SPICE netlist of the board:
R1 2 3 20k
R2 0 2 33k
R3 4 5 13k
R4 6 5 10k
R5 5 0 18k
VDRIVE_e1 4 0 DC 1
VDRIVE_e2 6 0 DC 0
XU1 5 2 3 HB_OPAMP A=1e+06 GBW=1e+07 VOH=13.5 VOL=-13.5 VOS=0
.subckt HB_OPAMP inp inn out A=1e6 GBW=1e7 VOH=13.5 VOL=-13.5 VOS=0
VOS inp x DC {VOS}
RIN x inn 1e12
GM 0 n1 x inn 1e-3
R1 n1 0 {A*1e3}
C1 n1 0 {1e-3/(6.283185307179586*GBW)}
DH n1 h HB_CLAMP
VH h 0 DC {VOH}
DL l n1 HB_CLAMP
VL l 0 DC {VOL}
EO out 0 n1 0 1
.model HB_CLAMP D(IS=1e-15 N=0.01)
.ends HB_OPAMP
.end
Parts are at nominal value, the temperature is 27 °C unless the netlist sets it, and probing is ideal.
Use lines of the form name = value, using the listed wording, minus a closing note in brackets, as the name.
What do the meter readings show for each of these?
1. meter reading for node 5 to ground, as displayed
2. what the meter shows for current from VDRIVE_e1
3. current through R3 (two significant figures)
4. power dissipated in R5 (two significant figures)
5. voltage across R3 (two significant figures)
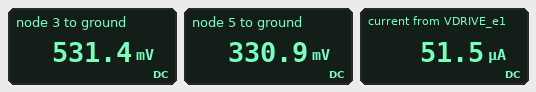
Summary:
meter reading for node 5 to ground, as displayed = 330.9 mV
what the meter shows for current from VDRIVE_e1 = 51.5 µA
current through R3 = 51 µA
power dissipated in R5 = 6.1 µW
voltage across R3 = 670 mV
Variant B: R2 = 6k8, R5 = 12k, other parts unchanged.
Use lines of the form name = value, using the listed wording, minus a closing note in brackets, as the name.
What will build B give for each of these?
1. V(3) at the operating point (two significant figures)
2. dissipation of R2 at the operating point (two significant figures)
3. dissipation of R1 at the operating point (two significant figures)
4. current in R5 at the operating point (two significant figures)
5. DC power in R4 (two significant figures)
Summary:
V(3) at the operating point = 1.2 V
dissipation of R2 at the operating point = 13 µW
dissipation of R1 at the operating point = 38 µW
current in R5 at the operating point = 25 µA
DC power in R4 = 8.7 µW
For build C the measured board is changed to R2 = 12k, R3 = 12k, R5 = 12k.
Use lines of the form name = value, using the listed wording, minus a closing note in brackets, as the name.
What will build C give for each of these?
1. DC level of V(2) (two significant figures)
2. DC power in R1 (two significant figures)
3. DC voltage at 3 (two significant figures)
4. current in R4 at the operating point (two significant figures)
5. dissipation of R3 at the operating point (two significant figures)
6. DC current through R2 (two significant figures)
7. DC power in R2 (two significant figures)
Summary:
DC level of V(2) = 310 mV
DC power in R1 = 14 µW
DC voltage at 3 = 830 mV
current in R4 at the operating point = 31 µA
dissipation of R3 at the operating point = 39 µW
DC current through R2 = 26 µA
DC power in R2 = 8.1 µW
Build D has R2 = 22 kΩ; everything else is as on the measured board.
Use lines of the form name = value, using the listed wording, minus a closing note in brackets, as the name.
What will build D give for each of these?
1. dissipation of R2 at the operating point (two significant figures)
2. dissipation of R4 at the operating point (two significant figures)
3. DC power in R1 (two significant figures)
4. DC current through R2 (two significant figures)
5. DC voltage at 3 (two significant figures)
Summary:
dissipation of R2 at the operating point = 5.0 µW
dissipation of R4 at the operating point = 11 µW
DC power in R1 = 4.5 µW
DC current through R2 = 15 µA
DC voltage at 3 = 630 mV
